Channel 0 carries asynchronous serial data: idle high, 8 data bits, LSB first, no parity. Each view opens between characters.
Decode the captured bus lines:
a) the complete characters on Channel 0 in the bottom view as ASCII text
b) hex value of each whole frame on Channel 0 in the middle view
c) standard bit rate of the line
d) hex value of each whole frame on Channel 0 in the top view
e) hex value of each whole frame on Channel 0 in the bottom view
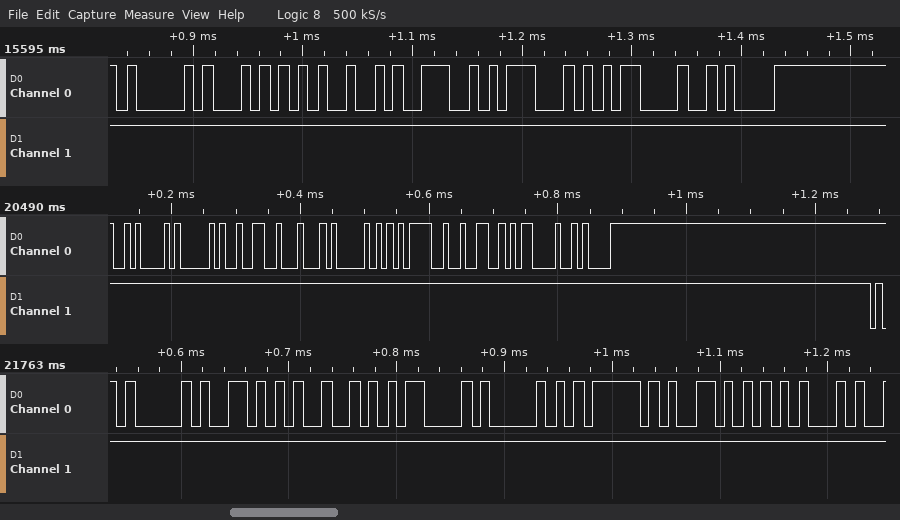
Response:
"AVRCP_VE"
0A, 41, 32, 44, 50, 3D, 32, 0D, 0A
115200 baud
41, 54, 49, 4E, 47, 0D, 0A
41, 56, 52, 43, 50, 5F, 56, 45
